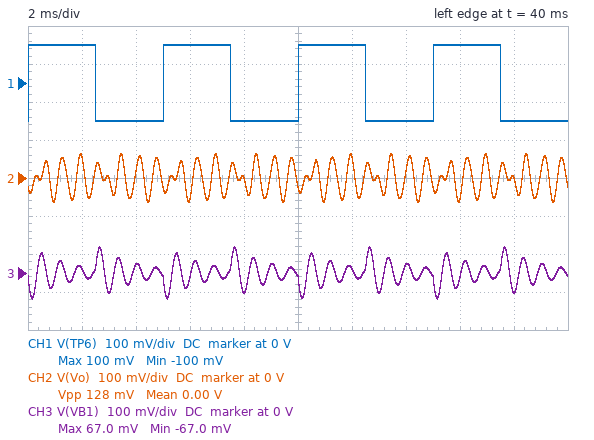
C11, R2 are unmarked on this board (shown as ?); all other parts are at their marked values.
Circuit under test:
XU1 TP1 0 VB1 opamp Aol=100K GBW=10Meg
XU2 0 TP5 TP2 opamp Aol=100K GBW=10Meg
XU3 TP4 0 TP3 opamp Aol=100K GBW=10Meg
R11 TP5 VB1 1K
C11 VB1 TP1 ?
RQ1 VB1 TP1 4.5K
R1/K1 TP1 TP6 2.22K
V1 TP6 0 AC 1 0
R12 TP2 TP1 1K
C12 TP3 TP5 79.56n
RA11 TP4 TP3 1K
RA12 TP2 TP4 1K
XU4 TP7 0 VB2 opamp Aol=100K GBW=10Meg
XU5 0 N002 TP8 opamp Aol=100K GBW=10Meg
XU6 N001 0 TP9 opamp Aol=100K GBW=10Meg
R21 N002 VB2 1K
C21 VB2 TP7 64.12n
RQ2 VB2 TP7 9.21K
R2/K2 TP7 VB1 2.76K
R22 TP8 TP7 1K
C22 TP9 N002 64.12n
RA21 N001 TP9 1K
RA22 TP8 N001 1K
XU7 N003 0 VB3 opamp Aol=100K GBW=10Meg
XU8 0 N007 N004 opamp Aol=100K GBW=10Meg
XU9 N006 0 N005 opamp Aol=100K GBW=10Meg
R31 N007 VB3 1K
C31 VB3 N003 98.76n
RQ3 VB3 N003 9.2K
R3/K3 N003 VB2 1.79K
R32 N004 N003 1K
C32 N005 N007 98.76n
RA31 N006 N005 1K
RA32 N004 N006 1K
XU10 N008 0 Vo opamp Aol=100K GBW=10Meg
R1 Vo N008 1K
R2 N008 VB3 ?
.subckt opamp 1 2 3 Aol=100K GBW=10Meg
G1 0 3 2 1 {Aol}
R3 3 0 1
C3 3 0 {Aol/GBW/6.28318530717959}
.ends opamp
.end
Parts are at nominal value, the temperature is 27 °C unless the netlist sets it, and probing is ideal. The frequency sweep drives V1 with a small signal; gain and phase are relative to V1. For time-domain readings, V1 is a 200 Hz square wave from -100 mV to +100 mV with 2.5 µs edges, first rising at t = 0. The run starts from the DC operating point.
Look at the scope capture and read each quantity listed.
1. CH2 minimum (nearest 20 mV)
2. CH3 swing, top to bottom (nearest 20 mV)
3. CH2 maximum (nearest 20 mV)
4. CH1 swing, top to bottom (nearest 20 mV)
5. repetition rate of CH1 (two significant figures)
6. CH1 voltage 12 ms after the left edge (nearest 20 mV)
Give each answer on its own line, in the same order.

-60 mV
140 mV
60 mV
200 mV
200 Hz
100 mV
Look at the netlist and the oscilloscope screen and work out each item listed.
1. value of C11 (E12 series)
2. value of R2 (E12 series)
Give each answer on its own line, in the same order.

150 nF
470 Ω
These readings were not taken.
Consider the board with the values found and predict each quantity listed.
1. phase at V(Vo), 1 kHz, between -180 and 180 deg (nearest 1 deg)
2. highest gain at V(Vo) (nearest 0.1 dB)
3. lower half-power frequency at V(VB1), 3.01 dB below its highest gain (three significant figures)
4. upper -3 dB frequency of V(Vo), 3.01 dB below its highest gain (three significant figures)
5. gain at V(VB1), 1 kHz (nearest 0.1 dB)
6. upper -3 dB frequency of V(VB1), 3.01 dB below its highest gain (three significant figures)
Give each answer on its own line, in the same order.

-111 deg
15.1 dB
1.34 kHz
1.67 kHz
-7.6 dB
1.58 kHz
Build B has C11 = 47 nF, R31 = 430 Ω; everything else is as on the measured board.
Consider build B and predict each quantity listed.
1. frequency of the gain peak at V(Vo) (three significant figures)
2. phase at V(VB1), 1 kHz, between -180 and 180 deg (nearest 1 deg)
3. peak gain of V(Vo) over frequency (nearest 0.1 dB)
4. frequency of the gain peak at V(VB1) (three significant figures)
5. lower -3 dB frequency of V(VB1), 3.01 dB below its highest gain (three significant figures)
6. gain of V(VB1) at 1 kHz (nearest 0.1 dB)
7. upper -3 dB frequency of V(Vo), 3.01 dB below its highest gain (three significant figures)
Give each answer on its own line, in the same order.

2.47 kHz
-97 deg
36.7 dB
2.60 kHz
2.25 kHz
-11.6 dB
2.54 kHz
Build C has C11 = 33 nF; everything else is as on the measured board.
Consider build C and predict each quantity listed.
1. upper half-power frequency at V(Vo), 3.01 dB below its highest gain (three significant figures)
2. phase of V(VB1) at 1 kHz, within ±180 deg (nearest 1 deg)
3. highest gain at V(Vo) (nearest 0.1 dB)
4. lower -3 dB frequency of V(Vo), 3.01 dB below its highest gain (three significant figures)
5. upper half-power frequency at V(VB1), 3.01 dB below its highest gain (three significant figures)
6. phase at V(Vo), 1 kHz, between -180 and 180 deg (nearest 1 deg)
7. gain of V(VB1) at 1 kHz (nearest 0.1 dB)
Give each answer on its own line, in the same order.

2.63 kHz
-97 deg
14.7 dB
2.35 kHz
3.69 kHz
-106 deg
-12.1 dB
